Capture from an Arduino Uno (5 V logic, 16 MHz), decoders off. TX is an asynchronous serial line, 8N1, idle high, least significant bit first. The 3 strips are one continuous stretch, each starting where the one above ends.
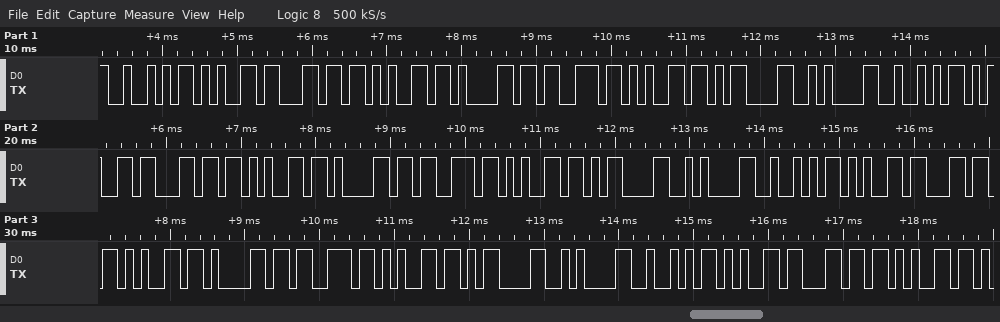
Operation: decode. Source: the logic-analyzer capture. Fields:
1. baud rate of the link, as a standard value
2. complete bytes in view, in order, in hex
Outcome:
9600 baud
52 65 6C 65 61 73 65 0D 0A 52 65 6C 65 61 73 65 0D 0A 52 65 6C 65 61 73 65 0D 0A 52 65 6C 65
